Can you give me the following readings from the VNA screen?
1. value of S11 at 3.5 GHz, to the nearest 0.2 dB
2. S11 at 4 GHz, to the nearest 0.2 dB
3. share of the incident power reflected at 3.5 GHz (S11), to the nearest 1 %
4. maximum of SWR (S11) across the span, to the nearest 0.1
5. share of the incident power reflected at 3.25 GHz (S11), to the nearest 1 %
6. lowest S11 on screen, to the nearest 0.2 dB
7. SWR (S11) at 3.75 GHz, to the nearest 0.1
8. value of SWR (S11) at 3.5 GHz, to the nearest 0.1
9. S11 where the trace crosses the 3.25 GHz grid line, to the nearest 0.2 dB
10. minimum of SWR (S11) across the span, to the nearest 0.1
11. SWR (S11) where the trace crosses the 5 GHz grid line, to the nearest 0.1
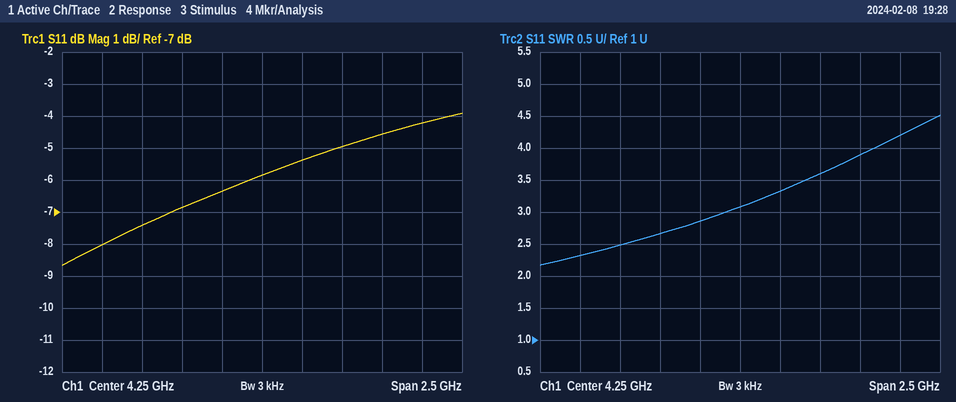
-7.4 dB
-6.4 dB
18 %
4.5
16 %
-8.6 dB
2.7
2.5
-8.0 dB
2.2
3.9
